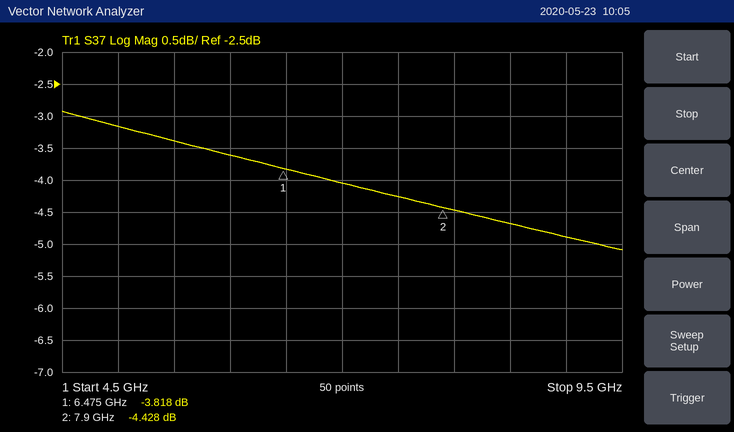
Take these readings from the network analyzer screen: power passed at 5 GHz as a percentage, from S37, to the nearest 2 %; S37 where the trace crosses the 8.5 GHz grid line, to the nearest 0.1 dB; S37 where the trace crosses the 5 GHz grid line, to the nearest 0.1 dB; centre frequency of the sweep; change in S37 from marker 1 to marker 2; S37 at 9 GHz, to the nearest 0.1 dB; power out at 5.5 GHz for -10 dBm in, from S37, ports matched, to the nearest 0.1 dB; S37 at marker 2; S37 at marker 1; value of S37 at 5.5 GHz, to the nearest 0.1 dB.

48 %
-4.7 dB
-3.2 dB
7 GHz
-0.610 dB
-4.9 dB
-13.4 dBm
-4.428 dB
-3.818 dB
-3.4 dB
